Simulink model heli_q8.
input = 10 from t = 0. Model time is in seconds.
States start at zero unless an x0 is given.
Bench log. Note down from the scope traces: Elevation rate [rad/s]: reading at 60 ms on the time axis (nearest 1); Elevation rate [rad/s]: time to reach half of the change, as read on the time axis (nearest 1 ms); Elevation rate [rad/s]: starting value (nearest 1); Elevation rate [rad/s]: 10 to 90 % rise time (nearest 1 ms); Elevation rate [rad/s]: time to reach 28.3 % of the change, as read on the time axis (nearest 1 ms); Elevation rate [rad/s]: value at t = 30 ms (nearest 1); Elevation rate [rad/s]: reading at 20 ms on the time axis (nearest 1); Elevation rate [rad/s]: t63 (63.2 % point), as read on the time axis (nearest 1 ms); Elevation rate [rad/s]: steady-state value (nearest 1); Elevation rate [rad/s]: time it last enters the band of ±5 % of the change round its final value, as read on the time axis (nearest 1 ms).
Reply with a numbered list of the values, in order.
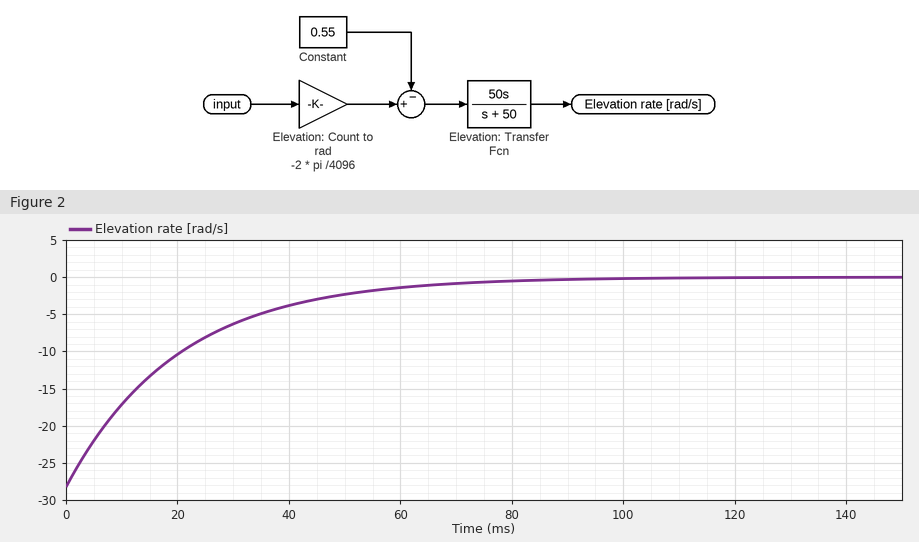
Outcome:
1. -1
2. 14 ms
3. -28
4. 44 ms
5. 7 ms
6. -6
7. -10
8. 20 ms
9. 0
10. 60 ms
